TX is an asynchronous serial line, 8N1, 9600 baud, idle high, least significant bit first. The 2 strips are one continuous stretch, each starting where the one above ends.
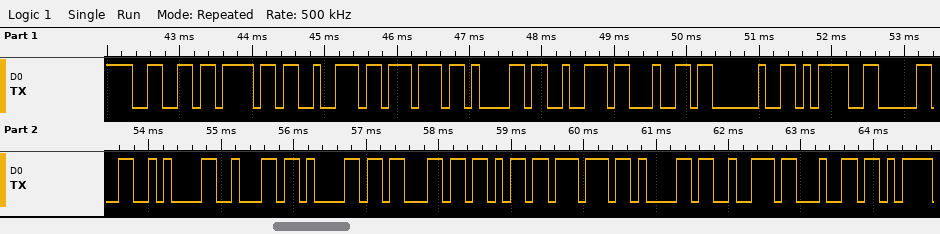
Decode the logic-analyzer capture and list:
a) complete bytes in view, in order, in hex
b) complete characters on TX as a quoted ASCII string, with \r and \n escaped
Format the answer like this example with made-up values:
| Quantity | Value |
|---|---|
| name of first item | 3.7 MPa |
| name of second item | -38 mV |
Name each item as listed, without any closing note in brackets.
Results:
| Quantity | Value |
|---|---|
| complete bytes in view, in order, in hex | 66 6F 72 77 61 72 64 20 3D 30 0A 62 61 63 6B 77 61 72 64 |
| complete characters on TX as a quoted ASCII string, with \r and \n escaped | "forward =0\nbackward" |
